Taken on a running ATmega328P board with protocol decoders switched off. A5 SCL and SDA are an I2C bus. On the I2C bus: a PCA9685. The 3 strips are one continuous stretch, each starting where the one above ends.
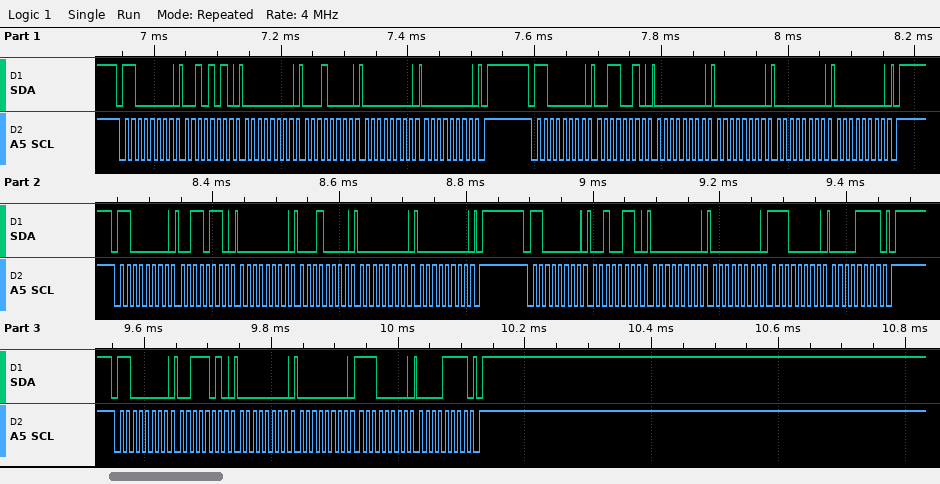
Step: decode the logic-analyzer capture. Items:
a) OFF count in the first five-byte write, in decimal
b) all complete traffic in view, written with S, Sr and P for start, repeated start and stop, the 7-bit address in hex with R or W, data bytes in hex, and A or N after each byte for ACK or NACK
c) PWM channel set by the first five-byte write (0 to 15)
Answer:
0
S 60W A 2A A 00 A 10 A 00 A 00 A P S 60W A 32 A 00 A 00 A 00 A 00 A P S 60W A 36 A 00 A 10 A 00 A 00 A P S 60W A 26 A 00 A 00 A E0 A 0F A P S 60W A 3A A 00 A 00 A E0 A 0F A P
9
